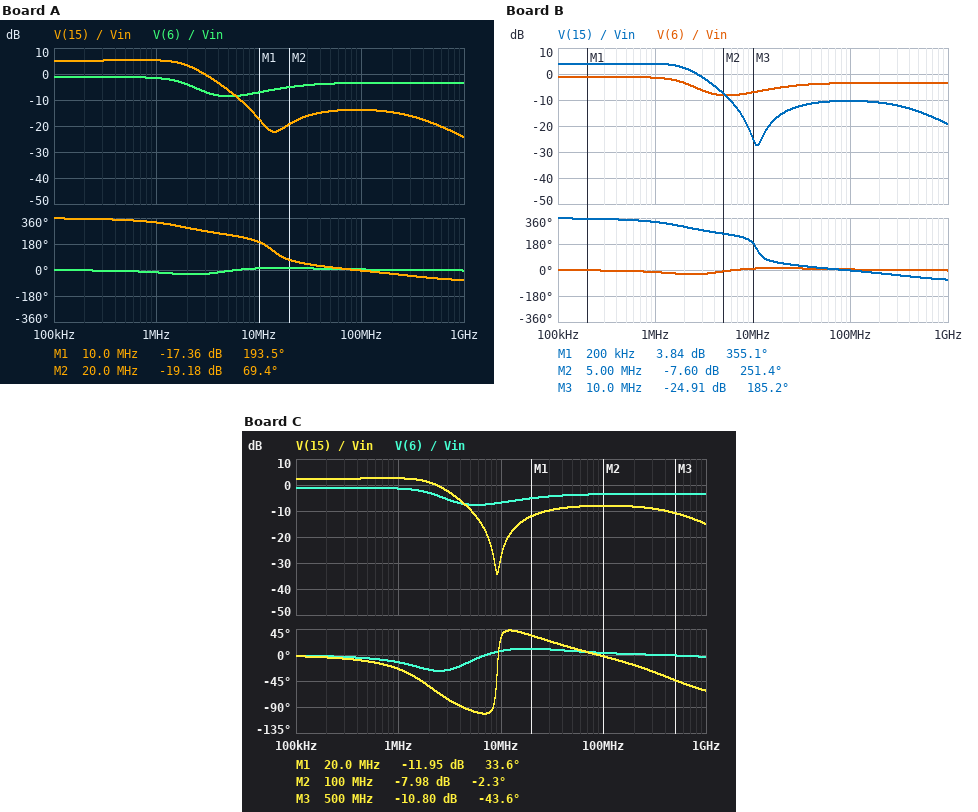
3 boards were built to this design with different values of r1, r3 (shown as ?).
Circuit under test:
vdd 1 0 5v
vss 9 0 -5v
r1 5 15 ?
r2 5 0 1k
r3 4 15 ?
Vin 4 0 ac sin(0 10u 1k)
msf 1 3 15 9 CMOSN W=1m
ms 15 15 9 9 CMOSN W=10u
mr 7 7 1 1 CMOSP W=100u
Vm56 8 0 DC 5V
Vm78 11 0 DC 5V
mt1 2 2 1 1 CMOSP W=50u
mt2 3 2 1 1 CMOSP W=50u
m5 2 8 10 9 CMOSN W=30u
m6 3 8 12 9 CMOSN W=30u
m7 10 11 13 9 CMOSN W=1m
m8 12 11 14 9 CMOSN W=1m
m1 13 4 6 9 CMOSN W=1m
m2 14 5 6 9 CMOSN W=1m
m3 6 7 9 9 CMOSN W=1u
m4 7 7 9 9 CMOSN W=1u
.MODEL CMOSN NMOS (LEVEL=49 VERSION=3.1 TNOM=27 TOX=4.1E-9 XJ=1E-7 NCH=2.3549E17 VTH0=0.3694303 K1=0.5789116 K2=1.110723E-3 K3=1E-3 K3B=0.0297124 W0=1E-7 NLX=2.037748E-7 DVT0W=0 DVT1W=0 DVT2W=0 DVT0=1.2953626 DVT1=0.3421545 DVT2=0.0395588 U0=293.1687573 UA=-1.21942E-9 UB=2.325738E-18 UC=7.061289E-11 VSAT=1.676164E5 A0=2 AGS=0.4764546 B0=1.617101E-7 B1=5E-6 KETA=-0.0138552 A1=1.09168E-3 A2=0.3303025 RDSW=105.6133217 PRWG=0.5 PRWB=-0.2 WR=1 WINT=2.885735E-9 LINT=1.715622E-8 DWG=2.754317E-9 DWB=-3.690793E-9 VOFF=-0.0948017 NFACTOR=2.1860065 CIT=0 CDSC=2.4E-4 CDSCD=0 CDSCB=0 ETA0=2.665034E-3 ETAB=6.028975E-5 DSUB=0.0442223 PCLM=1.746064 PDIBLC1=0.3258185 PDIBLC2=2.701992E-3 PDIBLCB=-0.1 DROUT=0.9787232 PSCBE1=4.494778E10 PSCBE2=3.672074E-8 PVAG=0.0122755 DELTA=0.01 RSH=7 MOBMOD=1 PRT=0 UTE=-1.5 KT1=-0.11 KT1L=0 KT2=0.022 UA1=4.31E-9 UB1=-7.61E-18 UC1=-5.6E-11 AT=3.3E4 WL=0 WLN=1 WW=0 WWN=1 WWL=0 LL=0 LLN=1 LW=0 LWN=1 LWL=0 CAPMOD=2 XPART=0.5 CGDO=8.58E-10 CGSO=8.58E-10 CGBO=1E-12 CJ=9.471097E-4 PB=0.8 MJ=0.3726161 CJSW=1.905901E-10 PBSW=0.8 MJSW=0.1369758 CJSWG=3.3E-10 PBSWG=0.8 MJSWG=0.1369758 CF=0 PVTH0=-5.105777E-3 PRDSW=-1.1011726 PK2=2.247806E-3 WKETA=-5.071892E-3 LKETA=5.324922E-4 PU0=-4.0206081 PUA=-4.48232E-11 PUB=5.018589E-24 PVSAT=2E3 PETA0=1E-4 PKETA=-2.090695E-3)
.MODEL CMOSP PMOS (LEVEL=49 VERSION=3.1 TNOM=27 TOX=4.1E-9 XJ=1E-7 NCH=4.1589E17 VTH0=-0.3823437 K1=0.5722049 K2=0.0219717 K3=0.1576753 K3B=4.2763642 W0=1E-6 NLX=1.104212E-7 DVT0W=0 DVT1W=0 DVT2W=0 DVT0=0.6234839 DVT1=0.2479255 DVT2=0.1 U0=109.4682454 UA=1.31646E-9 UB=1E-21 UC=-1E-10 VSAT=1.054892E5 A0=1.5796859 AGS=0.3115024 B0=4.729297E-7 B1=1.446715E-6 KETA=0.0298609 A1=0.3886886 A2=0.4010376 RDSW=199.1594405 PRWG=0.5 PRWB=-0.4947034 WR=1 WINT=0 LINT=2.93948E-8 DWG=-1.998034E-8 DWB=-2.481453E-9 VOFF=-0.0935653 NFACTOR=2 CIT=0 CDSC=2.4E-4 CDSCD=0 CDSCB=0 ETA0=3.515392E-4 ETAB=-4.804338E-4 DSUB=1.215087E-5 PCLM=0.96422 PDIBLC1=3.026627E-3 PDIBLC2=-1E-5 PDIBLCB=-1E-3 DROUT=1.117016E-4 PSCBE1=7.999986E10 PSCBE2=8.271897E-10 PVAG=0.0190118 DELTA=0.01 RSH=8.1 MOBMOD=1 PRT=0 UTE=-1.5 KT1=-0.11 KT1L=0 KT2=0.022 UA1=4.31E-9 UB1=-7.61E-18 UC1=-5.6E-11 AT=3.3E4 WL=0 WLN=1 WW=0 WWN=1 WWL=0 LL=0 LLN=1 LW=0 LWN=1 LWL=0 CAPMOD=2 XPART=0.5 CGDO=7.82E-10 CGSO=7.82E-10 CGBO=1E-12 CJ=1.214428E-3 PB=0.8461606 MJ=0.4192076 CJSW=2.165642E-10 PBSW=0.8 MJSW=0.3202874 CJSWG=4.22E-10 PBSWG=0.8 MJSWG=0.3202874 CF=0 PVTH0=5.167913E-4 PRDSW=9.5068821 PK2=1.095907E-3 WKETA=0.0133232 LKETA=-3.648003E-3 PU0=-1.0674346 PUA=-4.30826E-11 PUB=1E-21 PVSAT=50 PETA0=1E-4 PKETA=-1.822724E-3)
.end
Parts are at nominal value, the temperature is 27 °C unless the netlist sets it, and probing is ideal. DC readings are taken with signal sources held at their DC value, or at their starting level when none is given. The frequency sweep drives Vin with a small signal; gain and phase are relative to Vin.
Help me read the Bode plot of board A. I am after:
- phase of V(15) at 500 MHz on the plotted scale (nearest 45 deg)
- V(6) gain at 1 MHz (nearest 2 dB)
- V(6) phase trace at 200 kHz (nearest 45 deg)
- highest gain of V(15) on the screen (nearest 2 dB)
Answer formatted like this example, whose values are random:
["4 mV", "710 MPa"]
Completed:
["-45 deg", "-2 dB", "0 deg", "6 dB"]
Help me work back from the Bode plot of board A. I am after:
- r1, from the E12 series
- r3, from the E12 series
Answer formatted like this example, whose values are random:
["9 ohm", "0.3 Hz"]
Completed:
["820 Ω", "1.8 kΩ"]
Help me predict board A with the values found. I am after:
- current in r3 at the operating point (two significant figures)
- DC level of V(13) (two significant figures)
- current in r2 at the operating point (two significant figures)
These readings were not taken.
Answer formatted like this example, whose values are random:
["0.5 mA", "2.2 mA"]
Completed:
["4.8 µA", "3.1 V", "4.7 µA"]
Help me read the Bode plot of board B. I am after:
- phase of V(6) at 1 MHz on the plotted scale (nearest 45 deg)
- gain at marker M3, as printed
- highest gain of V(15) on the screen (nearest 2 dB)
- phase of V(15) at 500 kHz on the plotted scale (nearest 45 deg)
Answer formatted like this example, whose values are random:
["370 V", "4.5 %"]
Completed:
["0 deg", "-24.91 dB", "4 dB", "360 deg"]
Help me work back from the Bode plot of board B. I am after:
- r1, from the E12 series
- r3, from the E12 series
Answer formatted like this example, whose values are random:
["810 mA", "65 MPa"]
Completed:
["560 Ω", "820 Ω"]
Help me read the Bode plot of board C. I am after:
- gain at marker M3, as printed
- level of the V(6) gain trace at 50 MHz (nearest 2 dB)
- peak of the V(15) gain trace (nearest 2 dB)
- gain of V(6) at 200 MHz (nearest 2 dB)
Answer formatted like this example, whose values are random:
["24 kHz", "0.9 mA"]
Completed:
["-10.80 dB", "-4 dB", "2 dB", "-4 dB"]
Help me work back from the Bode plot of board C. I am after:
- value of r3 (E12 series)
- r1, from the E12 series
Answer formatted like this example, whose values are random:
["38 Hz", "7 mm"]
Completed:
["470 Ω", "330 Ω"]
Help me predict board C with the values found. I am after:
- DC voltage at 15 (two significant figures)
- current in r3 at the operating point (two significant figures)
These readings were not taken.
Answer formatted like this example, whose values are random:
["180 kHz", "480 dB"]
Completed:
["6.3 mV", "13 µA"]
